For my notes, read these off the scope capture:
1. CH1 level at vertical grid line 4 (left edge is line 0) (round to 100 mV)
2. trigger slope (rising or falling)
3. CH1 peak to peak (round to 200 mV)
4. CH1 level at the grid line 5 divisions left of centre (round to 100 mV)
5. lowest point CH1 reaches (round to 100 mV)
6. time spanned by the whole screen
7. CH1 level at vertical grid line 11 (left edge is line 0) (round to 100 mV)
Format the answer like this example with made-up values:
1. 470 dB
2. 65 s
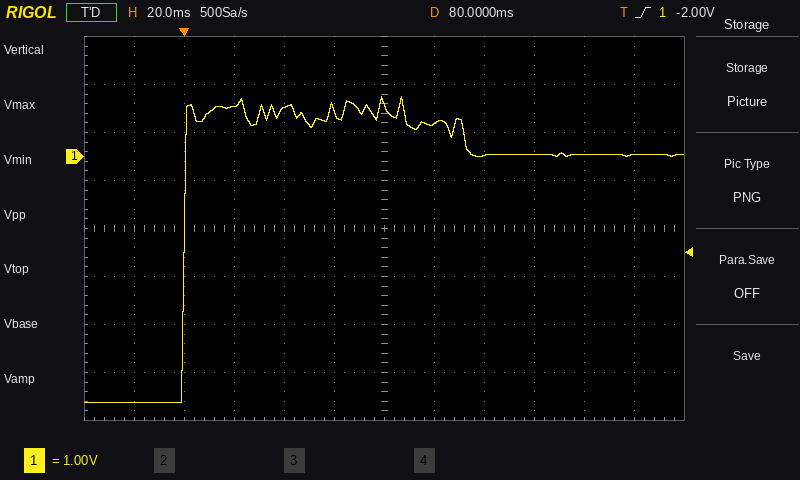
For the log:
1. 1.0 V
2. rising
3. 6.4 V
4. -5.1 V
5. -5.1 V
6. 240 ms
7. 0.0 V
